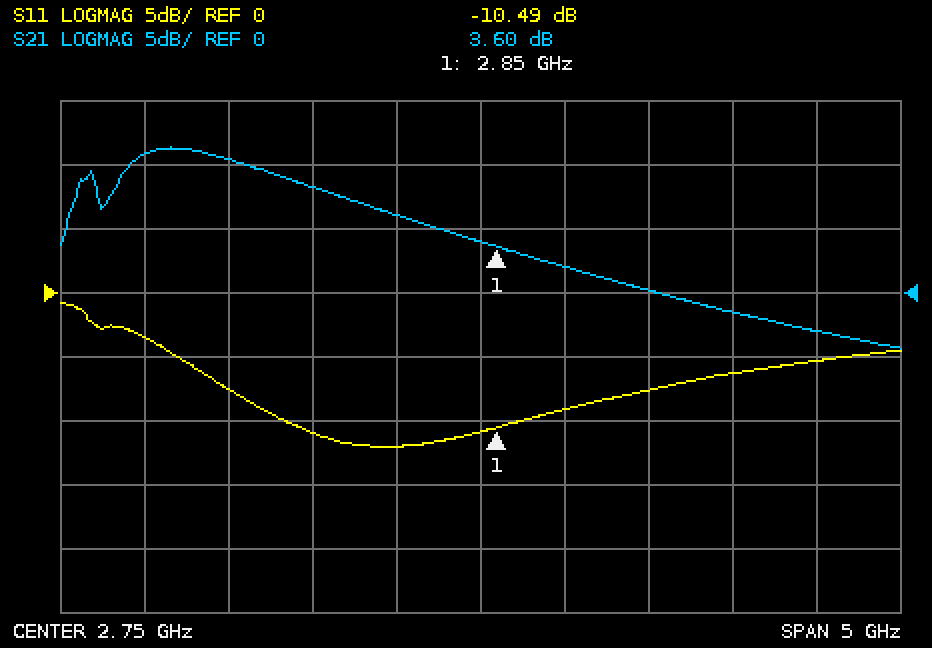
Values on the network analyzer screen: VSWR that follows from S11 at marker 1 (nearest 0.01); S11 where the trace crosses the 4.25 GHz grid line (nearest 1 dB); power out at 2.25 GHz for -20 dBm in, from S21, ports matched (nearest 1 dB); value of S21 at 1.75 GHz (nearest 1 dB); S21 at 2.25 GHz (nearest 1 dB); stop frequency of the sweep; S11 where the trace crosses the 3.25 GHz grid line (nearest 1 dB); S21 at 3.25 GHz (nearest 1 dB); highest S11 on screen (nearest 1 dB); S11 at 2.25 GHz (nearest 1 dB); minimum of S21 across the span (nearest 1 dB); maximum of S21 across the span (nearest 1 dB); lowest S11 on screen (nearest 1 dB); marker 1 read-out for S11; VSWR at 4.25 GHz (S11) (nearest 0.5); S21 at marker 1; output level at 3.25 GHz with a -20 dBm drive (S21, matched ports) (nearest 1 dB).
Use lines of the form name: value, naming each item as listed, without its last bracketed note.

VSWR that follows from S11 at marker 1: 1.85
S11 where the trace crosses the 4.25 GHz grid line: -6 dB
power out at 2.25 GHz for -20 dBm in, from S21, ports matched: -14 dBm
value of S21 at 1.75 GHz: 8 dB
S21 at 2.25 GHz: 6 dB
stop frequency of the sweep: 5.25 GHz
S11 where the trace crosses the 3.25 GHz grid line: -9 dB
S21 at 3.25 GHz: 2 dB
highest S11 on screen: -1 dB
S11 at 2.25 GHz: -12 dB
minimum of S21 across the span: -4 dB
maximum of S21 across the span: 11 dB
lowest S11 on screen: -12 dB
marker 1 read-out for S11: -10.49 dB
VSWR at 4.25 GHz (S11): 3.0
S21 at marker 1: 3.60 dB
output level at 3.25 GHz with a -20 dBm drive (S21, matched ports): -18 dBm
